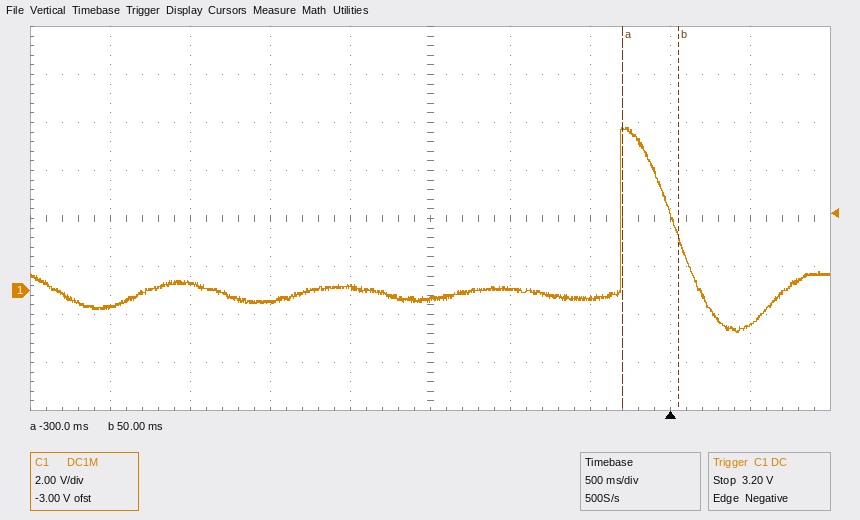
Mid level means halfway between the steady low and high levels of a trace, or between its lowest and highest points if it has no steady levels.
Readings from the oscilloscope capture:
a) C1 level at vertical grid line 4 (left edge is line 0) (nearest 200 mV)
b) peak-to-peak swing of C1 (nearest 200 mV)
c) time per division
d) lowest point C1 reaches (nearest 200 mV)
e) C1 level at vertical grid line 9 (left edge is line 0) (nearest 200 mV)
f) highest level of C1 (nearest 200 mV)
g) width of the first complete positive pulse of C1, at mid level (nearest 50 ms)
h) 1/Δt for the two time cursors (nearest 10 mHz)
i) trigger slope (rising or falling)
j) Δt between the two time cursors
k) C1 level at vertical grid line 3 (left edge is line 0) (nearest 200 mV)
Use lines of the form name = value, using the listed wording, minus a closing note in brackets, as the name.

C1 level at vertical grid line 4 (left edge is line 0) = 200 mV
peak-to-peak swing of C1 = 8.6 V
time per division = 500 ms
lowest point C1 reaches = -1.8 V
C1 level at vertical grid line 9 (left edge is line 0) = -1.4 V
highest level of C1 = 6.8 V
width of the first complete positive pulse of C1, at mid level = 350 ms
1/Δt for the two time cursors = 2.86 Hz
trigger slope = falling
Δt between the two time cursors = 350 ms
C1 level at vertical grid line 3 (left edge is line 0) = -400 mV
